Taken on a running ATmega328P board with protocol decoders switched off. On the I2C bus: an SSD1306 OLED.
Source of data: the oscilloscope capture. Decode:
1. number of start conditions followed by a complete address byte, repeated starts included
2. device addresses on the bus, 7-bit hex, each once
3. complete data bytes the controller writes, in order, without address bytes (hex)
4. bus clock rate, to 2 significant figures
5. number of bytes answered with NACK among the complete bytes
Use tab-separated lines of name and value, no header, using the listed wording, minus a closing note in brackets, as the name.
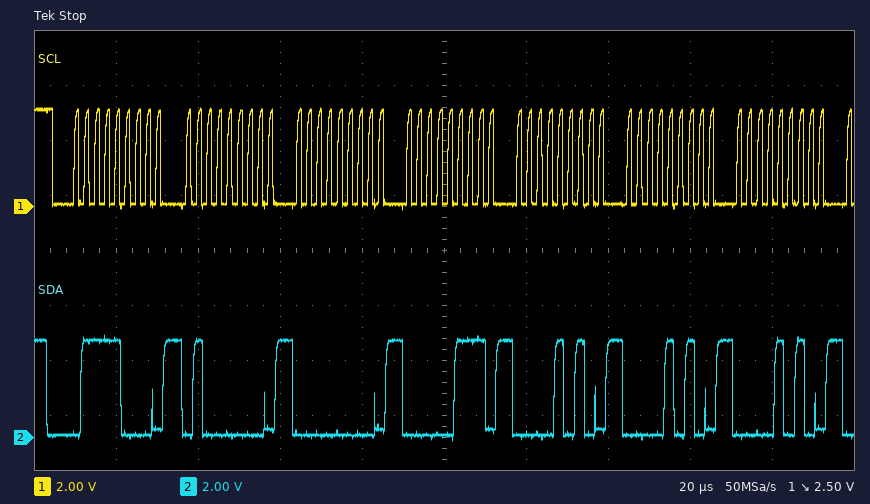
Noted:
number of start conditions followed by a complete address byte, repeated starts included	1
device addresses on the bus, 7-bit hex, each once	0x3C
complete data bytes the controller writes, in order, without address bytes	40 00 07 0A 0A 0A
bus clock rate, to 2 significant figures	400 kHz
number of bytes answered with NACK among the complete bytes	0
